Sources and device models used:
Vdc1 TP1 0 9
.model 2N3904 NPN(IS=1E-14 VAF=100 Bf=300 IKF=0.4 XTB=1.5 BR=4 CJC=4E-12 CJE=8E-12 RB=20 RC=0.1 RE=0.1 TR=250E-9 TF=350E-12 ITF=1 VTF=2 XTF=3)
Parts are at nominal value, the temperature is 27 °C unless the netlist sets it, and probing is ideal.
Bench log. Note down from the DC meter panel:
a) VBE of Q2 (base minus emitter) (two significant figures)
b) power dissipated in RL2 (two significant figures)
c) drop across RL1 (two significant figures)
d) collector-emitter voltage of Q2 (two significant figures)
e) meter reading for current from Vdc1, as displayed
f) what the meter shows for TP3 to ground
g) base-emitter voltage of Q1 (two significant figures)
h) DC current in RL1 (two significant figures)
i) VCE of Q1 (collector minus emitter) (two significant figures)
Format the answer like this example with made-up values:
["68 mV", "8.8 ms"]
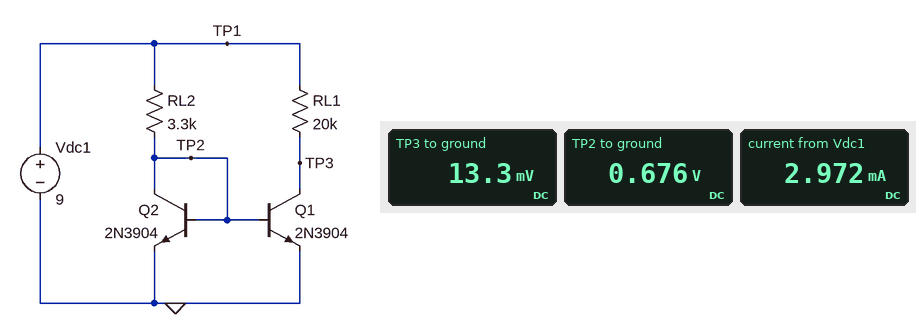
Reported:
["680 mV", "21 mW", "9.0 V", "680 mV", "2.972 mA", "13.3 mV", "680 mV", "450 µA", "13 mV"]
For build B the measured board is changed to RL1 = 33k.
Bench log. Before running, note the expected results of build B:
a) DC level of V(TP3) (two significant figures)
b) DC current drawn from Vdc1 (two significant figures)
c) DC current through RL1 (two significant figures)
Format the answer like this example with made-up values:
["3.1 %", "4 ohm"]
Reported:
["10 mV", "2.8 mA", "270 µA"]
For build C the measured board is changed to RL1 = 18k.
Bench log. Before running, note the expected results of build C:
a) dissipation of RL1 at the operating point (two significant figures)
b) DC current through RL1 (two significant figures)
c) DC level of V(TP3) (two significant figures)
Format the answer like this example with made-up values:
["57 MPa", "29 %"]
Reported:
["4.5 mW", "500 µA", "14 mV"]
